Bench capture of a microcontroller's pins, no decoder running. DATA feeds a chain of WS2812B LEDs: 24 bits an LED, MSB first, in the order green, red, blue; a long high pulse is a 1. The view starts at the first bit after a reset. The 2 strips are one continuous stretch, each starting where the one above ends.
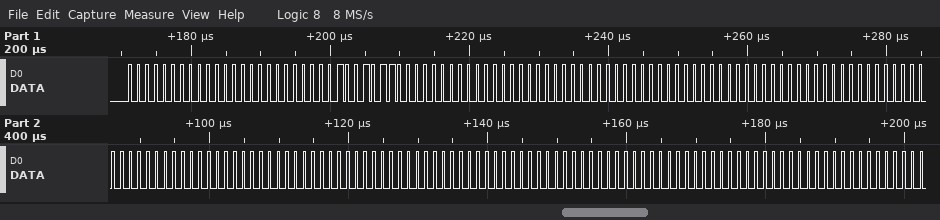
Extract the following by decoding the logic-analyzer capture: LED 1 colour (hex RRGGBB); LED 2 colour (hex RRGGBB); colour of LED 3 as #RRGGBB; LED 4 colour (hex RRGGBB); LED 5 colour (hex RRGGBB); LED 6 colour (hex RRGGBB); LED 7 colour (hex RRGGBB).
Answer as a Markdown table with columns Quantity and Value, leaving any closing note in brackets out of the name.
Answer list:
| Quantity | Value |
|---|---|
| LED 1 colour | #000000 |
| LED 2 colour | #009600 |
| colour of LED 3 as #RRGGBB | #000000 |
| LED 4 colour | #000000 |
| LED 5 colour | #000000 |
| LED 6 colour | #000000 |
| LED 7 colour | #000000 |
